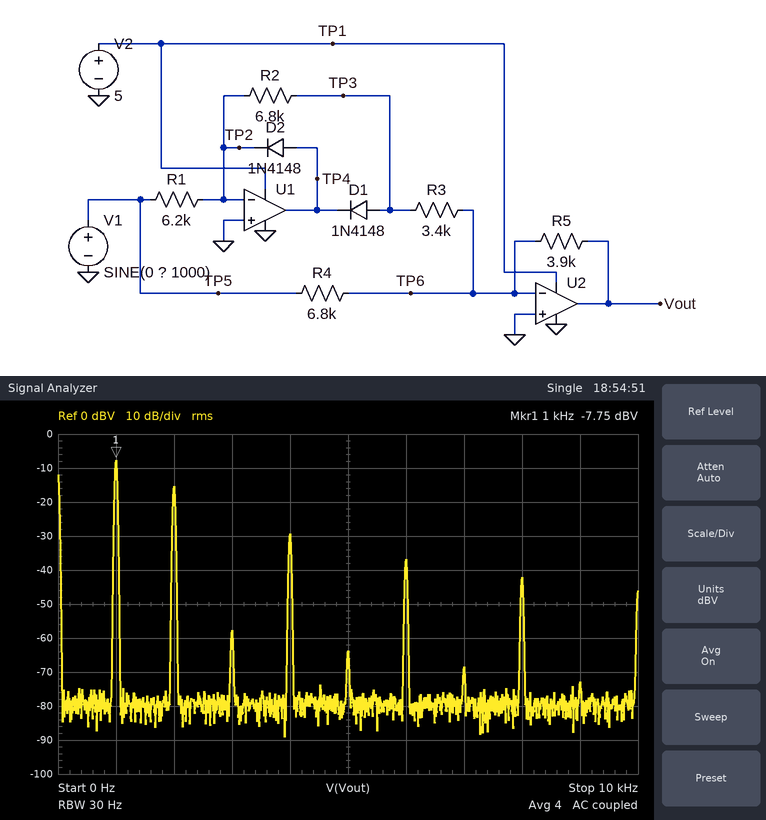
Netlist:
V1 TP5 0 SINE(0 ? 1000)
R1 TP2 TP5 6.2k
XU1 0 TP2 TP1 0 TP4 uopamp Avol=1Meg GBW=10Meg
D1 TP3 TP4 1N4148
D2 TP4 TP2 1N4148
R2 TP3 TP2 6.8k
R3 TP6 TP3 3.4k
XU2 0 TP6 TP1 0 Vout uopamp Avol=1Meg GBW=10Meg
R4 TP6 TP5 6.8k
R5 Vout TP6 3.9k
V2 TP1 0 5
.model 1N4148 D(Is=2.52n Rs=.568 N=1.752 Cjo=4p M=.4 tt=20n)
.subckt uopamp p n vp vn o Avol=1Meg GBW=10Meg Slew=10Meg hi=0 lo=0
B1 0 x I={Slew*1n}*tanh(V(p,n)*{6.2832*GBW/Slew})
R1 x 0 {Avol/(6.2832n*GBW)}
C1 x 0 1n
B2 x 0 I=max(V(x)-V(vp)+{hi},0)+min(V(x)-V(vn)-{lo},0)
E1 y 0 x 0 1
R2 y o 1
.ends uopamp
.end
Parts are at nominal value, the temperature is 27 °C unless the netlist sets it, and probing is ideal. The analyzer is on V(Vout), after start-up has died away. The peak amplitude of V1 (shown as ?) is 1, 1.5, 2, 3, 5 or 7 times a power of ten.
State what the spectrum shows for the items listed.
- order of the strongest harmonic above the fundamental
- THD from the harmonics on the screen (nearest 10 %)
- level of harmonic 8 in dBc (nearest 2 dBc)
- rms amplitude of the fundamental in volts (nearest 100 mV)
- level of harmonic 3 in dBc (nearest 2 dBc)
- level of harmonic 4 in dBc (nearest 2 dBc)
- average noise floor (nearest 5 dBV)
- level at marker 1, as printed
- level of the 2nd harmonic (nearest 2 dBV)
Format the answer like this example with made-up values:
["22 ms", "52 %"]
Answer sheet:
["2", "40 %", "-34 dBc", "400 mV", "-50 dBc", "-22 dBc", "-80 dBV", "-7.75 dBV", "-16 dBV"]
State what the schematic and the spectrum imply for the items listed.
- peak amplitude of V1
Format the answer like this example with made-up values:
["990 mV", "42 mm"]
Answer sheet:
["2 V"]
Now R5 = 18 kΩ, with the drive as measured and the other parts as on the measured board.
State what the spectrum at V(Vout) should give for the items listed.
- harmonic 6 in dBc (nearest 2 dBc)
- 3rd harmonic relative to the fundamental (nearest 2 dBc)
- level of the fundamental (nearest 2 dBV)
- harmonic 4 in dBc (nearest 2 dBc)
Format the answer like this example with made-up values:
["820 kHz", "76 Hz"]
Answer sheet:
["-32 dBc", "-36 dBc", "6 dBV", "-20 dBc"]
